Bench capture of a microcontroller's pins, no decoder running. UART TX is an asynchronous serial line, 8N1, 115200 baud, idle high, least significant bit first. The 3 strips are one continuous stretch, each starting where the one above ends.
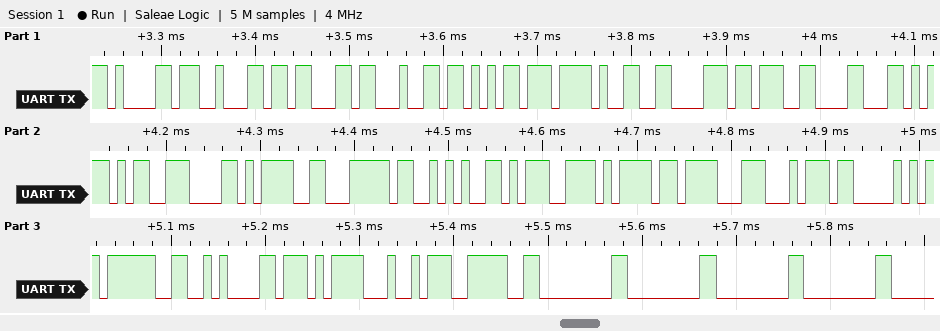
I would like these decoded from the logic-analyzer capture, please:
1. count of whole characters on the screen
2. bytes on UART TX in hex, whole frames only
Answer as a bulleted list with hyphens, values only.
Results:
- 28
- 0x61 0x62 0x63 0x64 0xB5 0x2F 0x86 0x3B 0x18 0x5D 0x0E 0x3D 0x7C 0x2A 0x9D 0xBD 0x8F 0x74 0x50 0x3F 0x0A 0xD7 0xA4 0x3E 0x00 0x00 0x00 0x00
